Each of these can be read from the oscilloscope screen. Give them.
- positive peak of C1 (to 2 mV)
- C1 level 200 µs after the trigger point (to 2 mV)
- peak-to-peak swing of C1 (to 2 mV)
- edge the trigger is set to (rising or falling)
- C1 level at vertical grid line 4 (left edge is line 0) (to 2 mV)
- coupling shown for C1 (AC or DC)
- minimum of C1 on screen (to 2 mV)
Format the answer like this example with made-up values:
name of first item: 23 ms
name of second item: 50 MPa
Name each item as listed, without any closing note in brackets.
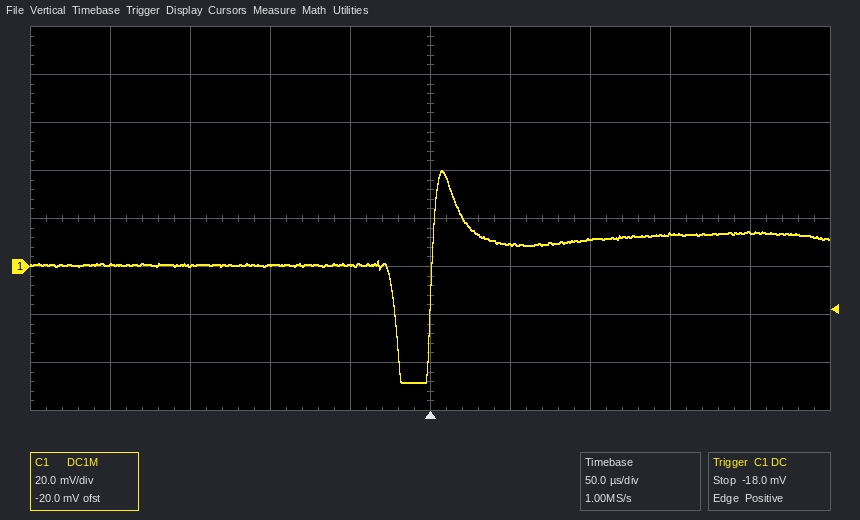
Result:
positive peak of C1: 40 mV
C1 level 200 µs after the trigger point: 14 mV
peak-to-peak swing of C1: 88 mV
edge the trigger is set to: rising
C1 level at vertical grid line 4 (left edge is line 0): 0 mV
coupling shown for C1: DC
minimum of C1 on screen: -48 mV
